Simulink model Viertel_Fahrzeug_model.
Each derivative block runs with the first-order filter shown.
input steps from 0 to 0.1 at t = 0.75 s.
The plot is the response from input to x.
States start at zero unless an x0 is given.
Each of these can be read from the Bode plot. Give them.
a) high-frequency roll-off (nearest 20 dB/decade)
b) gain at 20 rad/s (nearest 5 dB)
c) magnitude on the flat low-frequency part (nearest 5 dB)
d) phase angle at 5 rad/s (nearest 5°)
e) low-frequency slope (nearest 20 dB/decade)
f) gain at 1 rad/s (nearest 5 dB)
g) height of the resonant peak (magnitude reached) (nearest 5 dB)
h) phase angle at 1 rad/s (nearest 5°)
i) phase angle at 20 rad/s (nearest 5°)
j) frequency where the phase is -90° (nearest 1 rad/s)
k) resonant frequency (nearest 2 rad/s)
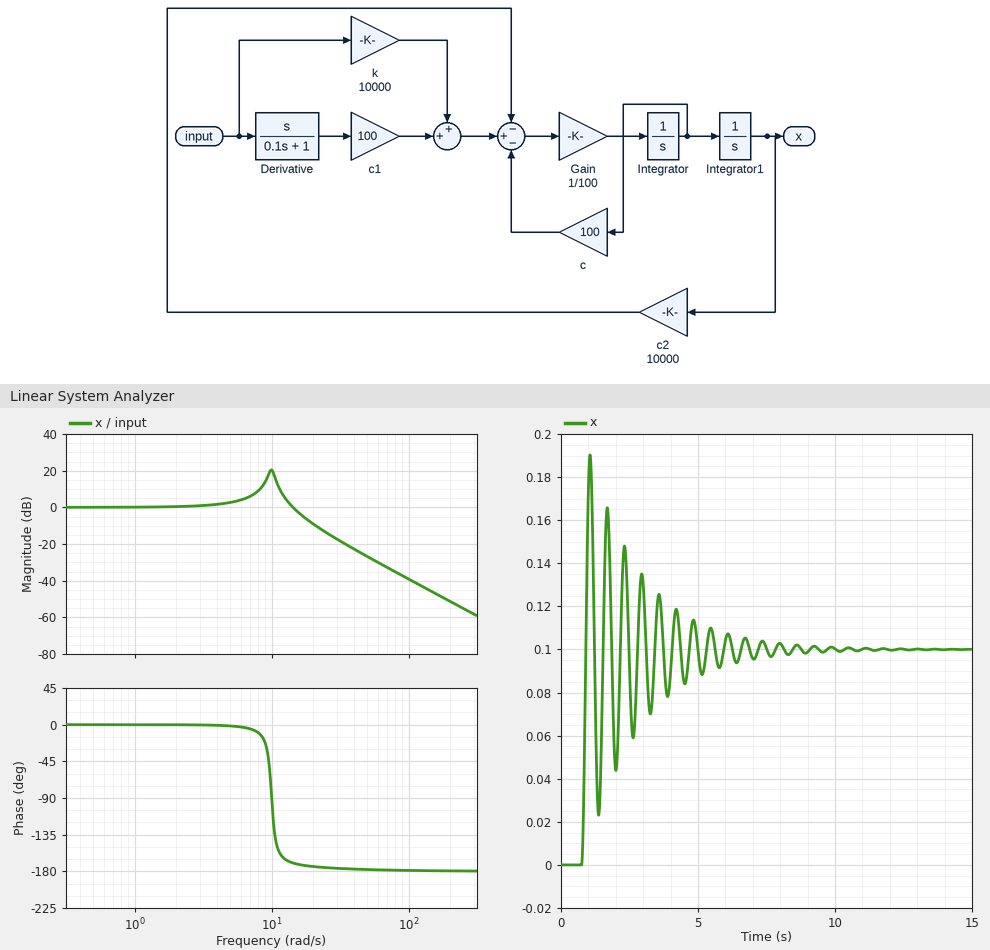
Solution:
-40 dB/decade
-10 dB
0 dB
0°
0 dB/decade
0 dB
20 dB
0°
-175°
10 rad/s
10 rad/s
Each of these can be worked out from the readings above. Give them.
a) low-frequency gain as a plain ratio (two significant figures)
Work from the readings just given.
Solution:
1.0
